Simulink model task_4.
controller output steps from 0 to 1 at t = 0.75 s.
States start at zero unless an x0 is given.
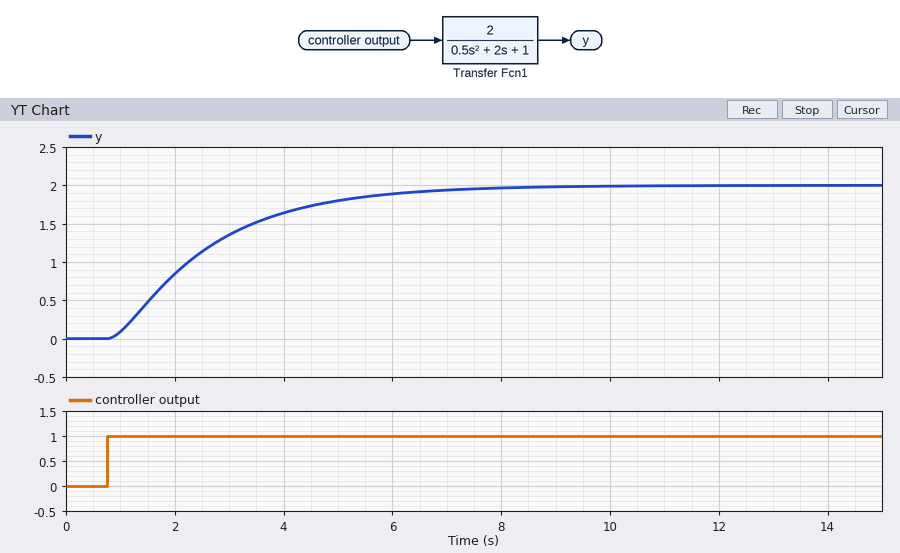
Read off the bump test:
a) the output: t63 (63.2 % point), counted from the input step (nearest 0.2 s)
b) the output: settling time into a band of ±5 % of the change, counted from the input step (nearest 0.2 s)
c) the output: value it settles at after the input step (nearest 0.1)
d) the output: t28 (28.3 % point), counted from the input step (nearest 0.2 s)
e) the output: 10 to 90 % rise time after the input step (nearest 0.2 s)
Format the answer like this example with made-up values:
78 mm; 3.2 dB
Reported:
2.0 s; 5.4 s; 2.0; 0.8 s; 3.8 s
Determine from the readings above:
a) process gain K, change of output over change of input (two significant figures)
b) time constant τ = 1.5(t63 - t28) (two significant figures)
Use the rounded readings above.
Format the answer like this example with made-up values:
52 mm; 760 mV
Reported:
2.0; 1.8 s
